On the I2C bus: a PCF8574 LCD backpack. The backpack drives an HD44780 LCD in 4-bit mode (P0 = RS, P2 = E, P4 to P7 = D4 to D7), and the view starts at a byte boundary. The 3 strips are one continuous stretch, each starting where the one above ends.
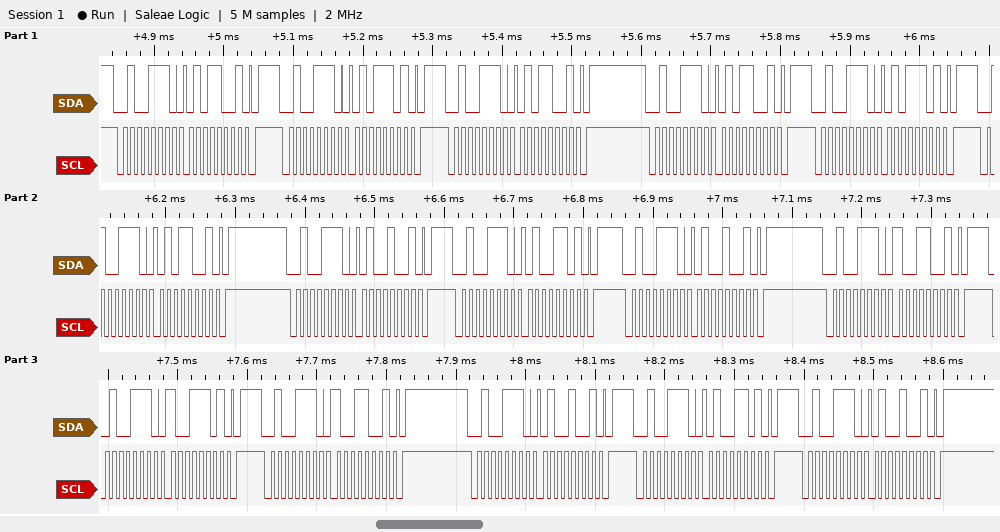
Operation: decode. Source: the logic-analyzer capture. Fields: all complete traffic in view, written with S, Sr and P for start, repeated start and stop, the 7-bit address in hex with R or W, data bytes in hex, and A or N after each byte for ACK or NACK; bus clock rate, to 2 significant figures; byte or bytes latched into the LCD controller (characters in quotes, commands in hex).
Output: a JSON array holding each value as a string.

["S 27W A 59 A P S 27W A 5D A P S 27W A 59 A P S 27W A 59 A P S 27W A 5D A P S 27W A 59 A P S 27W A 49 A P S 27W A 4D A P S 27W A 49 A P S 27W A 99 A P S 27W A 9D A P S 27W A 99 A P S 27W A 49 A P S 27W A 4D A P S 27W A 49 A P", "100 kHz", "'U' 'I'"]
